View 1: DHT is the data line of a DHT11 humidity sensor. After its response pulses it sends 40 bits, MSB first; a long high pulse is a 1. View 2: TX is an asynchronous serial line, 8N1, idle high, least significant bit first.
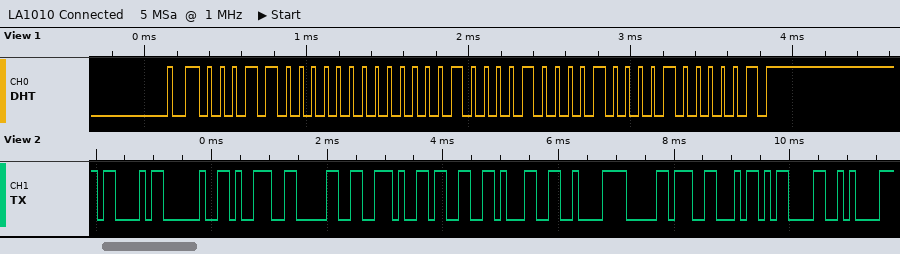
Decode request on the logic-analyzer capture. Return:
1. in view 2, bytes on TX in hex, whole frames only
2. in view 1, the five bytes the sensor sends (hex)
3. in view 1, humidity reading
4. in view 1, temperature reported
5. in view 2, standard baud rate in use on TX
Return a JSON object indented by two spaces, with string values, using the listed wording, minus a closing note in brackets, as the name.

{
  "in view 2, bytes on TX in hex, whole frames only": "43 20 39 30 2E 33 31 C2 B0 46 0D 0A",
  "in view 1, the five bytes the sensor sends": "18 00 21 08 41",
  "in view 1, humidity reading": "24 %",
  "in view 1, temperature reported": "33.8 °C",
  "in view 2, standard baud rate in use on TX": "9600 baud"
}
